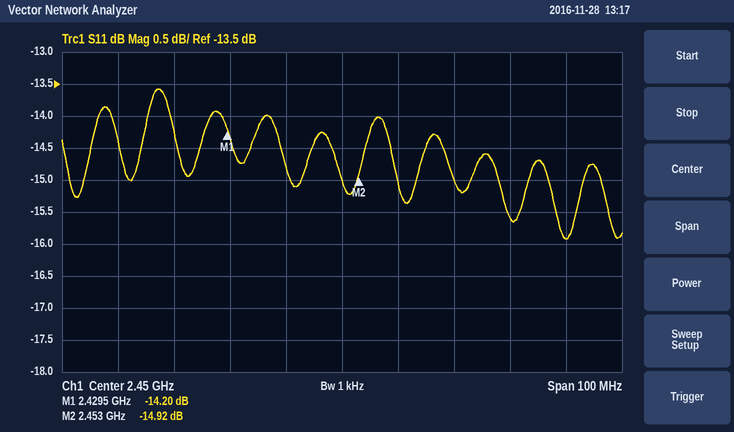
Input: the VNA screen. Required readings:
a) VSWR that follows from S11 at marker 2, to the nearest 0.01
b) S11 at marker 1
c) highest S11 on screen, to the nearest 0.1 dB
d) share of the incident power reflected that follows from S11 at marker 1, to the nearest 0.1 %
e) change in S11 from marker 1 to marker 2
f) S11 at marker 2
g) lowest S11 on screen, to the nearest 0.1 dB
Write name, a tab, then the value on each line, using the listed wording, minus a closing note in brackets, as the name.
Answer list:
VSWR that follows from S11 at marker 2, to the nearest 0.01	1.44
S11 at marker 1	-14.20 dB
highest S11 on screen, to the nearest 0.1 dB	-13.6 dB
share of the incident power reflected that follows from S11 at marker 1, to the nearest 0.1 %	3.8 %
change in S11 from marker 1 to marker 2	-0.72 dB
S11 at marker 2	-14.92 dB
lowest S11 on screen, to the nearest 0.1 dB	-15.9 dB
